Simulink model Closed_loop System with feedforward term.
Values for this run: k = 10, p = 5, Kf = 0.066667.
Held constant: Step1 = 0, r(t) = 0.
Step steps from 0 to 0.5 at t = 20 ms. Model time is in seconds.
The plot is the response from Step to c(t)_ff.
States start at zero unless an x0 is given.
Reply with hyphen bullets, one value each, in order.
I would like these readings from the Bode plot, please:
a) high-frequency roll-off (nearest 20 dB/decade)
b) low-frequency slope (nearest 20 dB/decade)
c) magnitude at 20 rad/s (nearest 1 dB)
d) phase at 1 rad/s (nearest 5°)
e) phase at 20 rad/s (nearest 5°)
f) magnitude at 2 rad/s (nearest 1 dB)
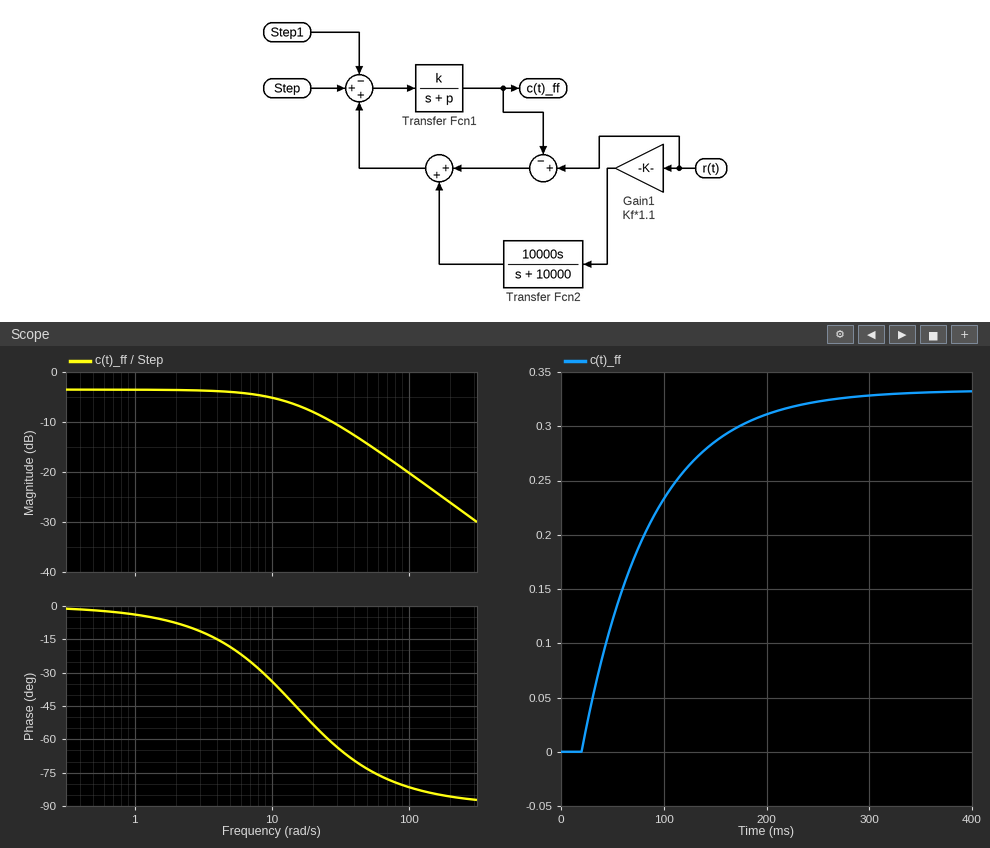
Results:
- -20 dB/decade
- 0 dB/decade
- -8 dB
- -5°
- -55°
- -4 dB
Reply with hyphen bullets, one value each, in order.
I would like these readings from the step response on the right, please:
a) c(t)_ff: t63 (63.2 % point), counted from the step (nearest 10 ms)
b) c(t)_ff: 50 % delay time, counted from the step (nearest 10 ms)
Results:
- 70 ms
- 50 ms
